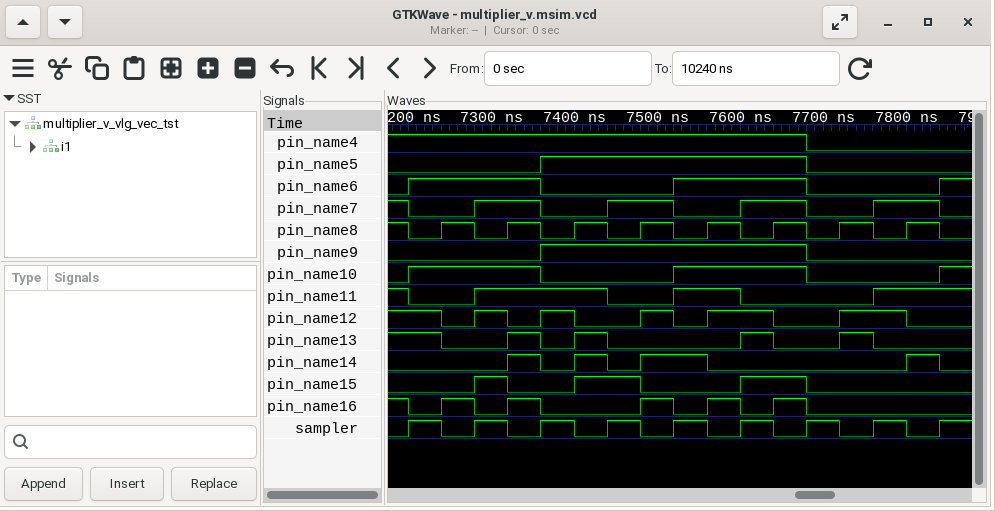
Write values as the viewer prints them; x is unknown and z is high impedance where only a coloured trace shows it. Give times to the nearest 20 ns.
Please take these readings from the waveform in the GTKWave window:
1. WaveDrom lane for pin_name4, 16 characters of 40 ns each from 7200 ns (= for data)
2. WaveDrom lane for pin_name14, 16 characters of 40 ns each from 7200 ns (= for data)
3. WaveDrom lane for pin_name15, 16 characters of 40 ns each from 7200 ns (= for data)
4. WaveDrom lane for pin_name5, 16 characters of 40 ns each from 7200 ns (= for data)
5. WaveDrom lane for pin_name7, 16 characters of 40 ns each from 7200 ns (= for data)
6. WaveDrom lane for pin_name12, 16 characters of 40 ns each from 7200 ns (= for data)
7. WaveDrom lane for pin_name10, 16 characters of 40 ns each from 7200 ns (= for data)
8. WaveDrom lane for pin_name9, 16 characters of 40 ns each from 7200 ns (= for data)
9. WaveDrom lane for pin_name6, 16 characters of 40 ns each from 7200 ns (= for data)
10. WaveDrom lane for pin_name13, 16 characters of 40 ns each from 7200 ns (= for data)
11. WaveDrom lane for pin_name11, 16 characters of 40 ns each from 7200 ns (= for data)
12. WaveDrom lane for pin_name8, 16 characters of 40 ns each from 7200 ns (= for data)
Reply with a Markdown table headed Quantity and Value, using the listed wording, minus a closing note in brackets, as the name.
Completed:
| Quantity | Value |
|---|---|
| WaveDrom lane for pin_name4, 16 characters of 40 ns each from 7200 ns | {name: 'pin_name4', wave: '1...........0...'} |
| WaveDrom lane for pin_name14, 16 characters of 40 ns each from 7200 ns | {name: 'pin_name14', wave: '0..10101.0.....1'} |
| WaveDrom lane for pin_name15, 16 characters of 40 ns each from 7200 ns | {name: 'pin_name15', wave: '0.10.1.0..1.0...'} |
| WaveDrom lane for pin_name5, 16 characters of 40 ns each from 7200 ns | {name: 'pin_name5', wave: '0...1.......0...'} |
| WaveDrom lane for pin_name7, 16 characters of 40 ns each from 7200 ns | {name: 'pin_name7', wave: '0.1.0.1.0.1.0.1.'} |
| WaveDrom lane for pin_name12, 16 characters of 40 ns each from 7200 ns | {name: 'pin_name12', wave: '101010.101.0.1.0'} |
| WaveDrom lane for pin_name10, 16 characters of 40 ns each from 7200 ns | {name: 'pin_name10', wave: '1...0...1...0...'} |
| WaveDrom lane for pin_name9, 16 characters of 40 ns each from 7200 ns | {name: 'pin_name9', wave: '0...1.......0...'} |
| WaveDrom lane for pin_name6, 16 characters of 40 ns each from 7200 ns | {name: 'pin_name6', wave: '1...0...1...0...'} |
| WaveDrom lane for pin_name13, 16 characters of 40 ns each from 7200 ns | {name: 'pin_name13', wave: '10.1010...10.10.'} |
| WaveDrom lane for pin_name11, 16 characters of 40 ns each from 7200 ns | {name: 'pin_name11', wave: '0.1...0.1.0...1.'} |
| WaveDrom lane for pin_name8, 16 characters of 40 ns each from 7200 ns | {name: 'pin_name8', wave: '0101010101010101'} |
